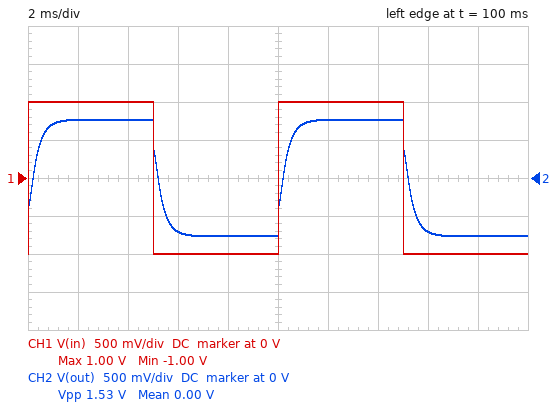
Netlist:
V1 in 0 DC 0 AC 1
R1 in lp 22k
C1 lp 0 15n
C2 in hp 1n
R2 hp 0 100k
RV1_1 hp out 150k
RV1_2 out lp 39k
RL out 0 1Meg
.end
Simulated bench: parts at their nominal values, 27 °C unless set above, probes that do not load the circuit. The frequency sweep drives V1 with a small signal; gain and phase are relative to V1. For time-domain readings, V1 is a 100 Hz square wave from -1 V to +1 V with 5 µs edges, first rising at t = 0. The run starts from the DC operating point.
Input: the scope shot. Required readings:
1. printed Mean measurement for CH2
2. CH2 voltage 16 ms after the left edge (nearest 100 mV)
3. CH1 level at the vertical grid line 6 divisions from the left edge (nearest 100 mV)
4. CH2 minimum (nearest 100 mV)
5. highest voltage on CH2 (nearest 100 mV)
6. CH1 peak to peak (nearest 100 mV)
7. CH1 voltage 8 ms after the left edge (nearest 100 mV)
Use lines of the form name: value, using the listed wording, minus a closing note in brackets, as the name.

printed Mean measurement for CH2: 0.00 V
CH2 voltage 16 ms after the left edge: -700 mV
CH1 level at the vertical grid line 6 divisions from the left edge: 1.0 V
CH2 minimum: -800 mV
highest voltage on CH2: 800 mV
CH1 peak to peak: 2.0 V
CH1 voltage 8 ms after the left edge: -1.0 V
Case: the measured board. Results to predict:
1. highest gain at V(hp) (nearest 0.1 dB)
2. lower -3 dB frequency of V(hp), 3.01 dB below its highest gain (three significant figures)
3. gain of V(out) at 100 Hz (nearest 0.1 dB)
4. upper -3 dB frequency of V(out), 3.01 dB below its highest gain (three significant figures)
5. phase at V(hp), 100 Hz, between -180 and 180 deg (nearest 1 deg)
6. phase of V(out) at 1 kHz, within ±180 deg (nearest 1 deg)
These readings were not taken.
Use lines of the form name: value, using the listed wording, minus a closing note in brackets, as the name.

highest gain at V(hp): 0 dB
lower -3 dB frequency of V(hp), 3.01 dB below its highest gain: 2.74 kHz
gain of V(out) at 100 Hz: -2.5 dB
upper -3 dB frequency of V(out), 3.01 dB below its highest gain: 487 Hz
phase at V(hp), 100 Hz, between -180 and 180 deg: -5 deg
phase of V(out) at 1 kHz, within ±180 deg: -51 deg
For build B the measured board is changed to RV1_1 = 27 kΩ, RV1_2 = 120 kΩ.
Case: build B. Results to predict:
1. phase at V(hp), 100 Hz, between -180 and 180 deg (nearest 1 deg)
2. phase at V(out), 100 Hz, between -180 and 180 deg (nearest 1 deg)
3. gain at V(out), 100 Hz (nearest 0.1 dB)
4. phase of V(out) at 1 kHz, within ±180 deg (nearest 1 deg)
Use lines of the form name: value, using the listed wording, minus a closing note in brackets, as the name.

phase at V(hp), 100 Hz, between -180 and 180 deg: -7 deg
phase at V(out), 100 Hz, between -180 and 180 deg: -8 deg
gain at V(out), 100 Hz: -7.3 dB
phase of V(out) at 1 kHz, within ±180 deg: 23 deg
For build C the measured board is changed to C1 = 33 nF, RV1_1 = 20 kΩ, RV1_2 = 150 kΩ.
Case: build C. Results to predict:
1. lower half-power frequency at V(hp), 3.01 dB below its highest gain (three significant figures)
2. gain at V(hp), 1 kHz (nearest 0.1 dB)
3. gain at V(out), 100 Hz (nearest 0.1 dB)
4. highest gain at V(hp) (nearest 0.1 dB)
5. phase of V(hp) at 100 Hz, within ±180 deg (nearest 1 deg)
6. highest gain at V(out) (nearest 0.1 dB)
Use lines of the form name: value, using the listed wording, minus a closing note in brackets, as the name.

lower half-power frequency at V(hp), 3.01 dB below its highest gain: 2.80 kHz
gain at V(hp), 1 kHz: -10.9 dB
gain at V(out), 100 Hz: -9.3 dB
highest gain at V(hp): 0 dB
phase of V(hp) at 100 Hz, within ±180 deg: -18 deg
highest gain at V(out): -1.2 dB
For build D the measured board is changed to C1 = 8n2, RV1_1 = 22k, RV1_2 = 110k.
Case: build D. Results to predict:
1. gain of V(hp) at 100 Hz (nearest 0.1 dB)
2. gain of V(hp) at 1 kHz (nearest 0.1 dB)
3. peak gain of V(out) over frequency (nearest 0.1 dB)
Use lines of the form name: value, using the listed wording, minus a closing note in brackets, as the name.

gain of V(hp) at 100 Hz: -8.7 dB
gain of V(hp) at 1 kHz: -12.5 dB
peak gain of V(out) over frequency: -1.7 dB
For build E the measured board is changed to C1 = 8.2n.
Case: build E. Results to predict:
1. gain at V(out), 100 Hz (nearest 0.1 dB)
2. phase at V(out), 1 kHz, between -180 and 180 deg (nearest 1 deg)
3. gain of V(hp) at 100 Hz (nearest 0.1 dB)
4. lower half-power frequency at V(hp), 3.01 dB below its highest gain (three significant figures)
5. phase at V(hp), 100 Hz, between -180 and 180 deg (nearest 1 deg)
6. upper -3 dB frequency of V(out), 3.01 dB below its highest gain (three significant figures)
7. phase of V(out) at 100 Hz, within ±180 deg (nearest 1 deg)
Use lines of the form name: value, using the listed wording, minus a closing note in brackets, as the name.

gain at V(out), 100 Hz: -2.4 dB
phase at V(out), 1 kHz, between -180 and 180 deg: -38 deg
gain of V(hp) at 100 Hz: -10.4 dB
lower half-power frequency at V(hp), 3.01 dB below its highest gain: 2.92 kHz
phase at V(hp), 100 Hz, between -180 and 180 deg: 0 deg
upper -3 dB frequency of V(out), 3.01 dB below its highest gain: 881 Hz
phase of V(out) at 100 Hz, within ±180 deg: -5 deg
